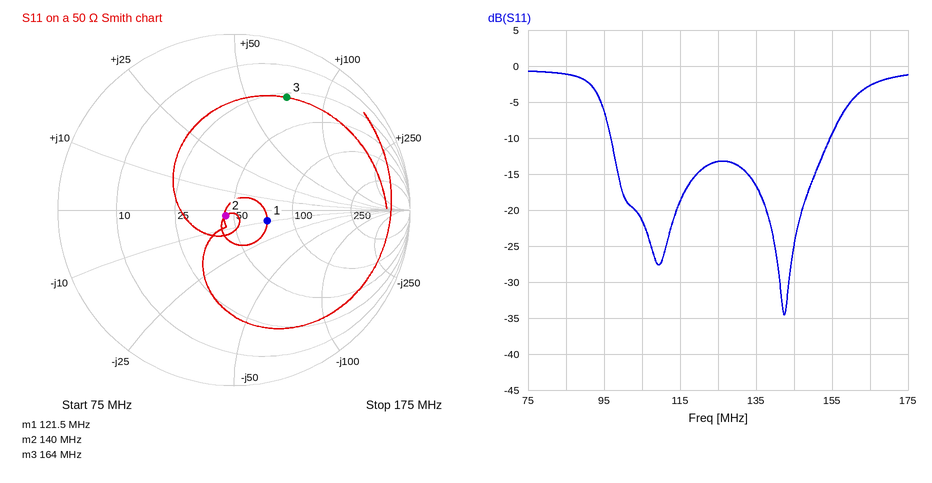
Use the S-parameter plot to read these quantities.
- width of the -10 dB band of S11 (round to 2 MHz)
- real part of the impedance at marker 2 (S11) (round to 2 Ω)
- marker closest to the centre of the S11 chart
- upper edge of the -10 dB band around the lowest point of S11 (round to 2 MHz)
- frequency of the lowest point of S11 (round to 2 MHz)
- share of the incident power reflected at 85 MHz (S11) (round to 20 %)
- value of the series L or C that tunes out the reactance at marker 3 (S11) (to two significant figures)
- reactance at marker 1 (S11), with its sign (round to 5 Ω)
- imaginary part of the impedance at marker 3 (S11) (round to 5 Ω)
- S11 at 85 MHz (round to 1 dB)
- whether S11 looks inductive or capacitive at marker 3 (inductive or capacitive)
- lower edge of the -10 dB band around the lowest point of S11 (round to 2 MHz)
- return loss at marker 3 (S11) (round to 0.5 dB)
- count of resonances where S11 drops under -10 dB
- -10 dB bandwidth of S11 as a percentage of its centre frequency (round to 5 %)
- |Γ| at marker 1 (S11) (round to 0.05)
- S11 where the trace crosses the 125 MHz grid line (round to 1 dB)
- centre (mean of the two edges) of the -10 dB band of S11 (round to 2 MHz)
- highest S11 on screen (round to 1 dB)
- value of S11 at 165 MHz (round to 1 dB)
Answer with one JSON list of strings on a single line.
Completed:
["58 MHz", "46 Ω", "marker 2", "154 MHz", "142 MHz", "80 %", "14 pF", "-10 Ω", "+70 Ω", "-1 dB", "inductive", "96 MHz", "3.0 dB", "2", "45 %", "0.20", "-13 dB", "126 MHz", "-1 dB", "-3 dB"]
